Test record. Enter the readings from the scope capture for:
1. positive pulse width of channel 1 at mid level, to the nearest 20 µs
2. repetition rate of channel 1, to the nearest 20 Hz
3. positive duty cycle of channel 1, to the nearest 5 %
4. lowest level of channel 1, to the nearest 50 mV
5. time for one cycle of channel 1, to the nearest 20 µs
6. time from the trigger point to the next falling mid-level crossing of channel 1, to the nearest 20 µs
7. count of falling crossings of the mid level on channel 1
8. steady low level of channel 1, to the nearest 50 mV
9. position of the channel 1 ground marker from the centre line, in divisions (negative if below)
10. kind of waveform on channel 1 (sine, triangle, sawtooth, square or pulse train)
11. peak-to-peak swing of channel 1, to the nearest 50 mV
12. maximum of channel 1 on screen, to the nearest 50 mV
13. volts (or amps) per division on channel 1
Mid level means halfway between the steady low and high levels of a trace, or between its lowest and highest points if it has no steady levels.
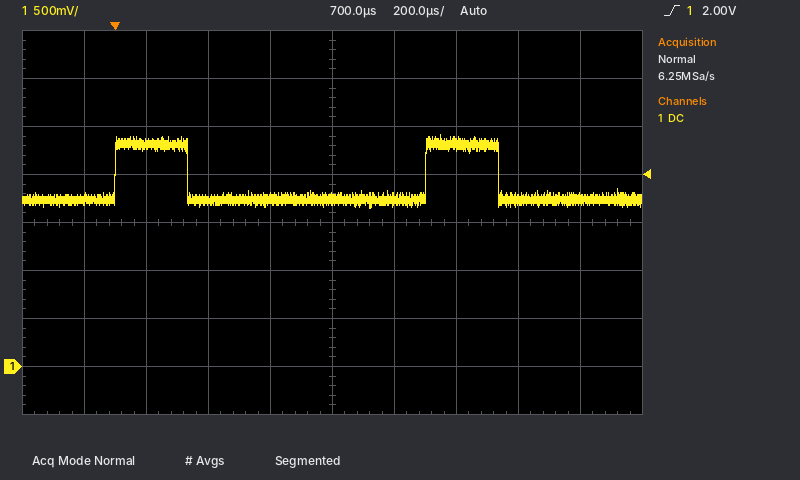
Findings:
240 µs
1.00 kHz
25 %
1.65 V
1.00 ms
240 µs
2
1.75 V
-3.0 div
pulse train
750 mV
2.40 V
500 mV
